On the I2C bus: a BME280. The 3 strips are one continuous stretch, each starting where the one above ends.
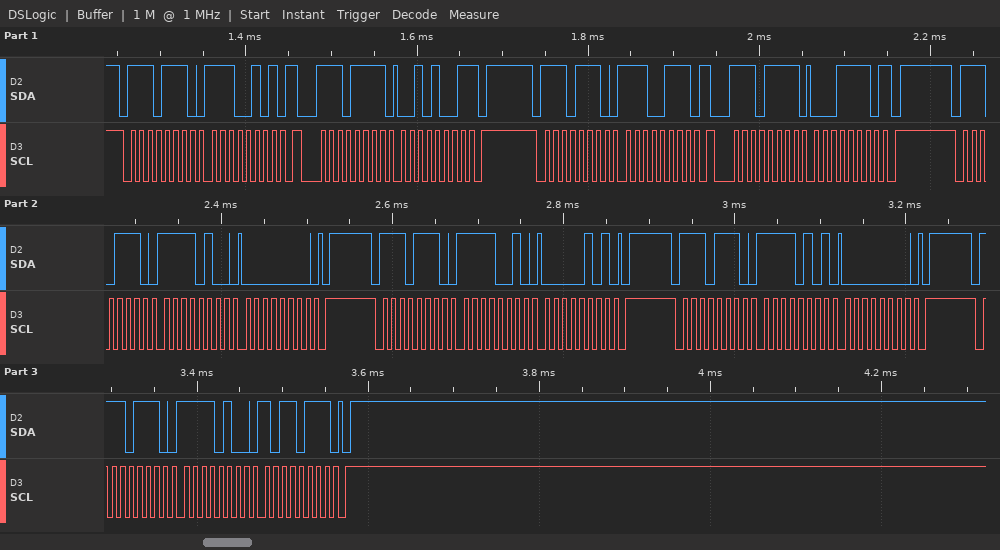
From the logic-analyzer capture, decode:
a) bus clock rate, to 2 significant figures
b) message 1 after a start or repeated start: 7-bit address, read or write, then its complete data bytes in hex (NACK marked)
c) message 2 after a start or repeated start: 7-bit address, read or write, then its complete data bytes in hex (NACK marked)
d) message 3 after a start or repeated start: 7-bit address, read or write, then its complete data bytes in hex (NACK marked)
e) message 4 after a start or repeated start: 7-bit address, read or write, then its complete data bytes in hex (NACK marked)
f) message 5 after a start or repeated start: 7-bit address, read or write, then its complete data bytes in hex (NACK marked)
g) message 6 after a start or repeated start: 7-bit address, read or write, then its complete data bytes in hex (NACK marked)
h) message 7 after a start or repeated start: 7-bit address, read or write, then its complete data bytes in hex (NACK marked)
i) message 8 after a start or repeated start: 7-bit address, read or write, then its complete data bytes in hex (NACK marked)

100 kHz
0x77 write: E5
0x77 read: 29 NACK
0x77 write: E7
0x77 read: 1E NACK
0x77 write: F4 00
0x77 write: F2 05
0x77 write: F5 00
0x77 write: F4 B7
